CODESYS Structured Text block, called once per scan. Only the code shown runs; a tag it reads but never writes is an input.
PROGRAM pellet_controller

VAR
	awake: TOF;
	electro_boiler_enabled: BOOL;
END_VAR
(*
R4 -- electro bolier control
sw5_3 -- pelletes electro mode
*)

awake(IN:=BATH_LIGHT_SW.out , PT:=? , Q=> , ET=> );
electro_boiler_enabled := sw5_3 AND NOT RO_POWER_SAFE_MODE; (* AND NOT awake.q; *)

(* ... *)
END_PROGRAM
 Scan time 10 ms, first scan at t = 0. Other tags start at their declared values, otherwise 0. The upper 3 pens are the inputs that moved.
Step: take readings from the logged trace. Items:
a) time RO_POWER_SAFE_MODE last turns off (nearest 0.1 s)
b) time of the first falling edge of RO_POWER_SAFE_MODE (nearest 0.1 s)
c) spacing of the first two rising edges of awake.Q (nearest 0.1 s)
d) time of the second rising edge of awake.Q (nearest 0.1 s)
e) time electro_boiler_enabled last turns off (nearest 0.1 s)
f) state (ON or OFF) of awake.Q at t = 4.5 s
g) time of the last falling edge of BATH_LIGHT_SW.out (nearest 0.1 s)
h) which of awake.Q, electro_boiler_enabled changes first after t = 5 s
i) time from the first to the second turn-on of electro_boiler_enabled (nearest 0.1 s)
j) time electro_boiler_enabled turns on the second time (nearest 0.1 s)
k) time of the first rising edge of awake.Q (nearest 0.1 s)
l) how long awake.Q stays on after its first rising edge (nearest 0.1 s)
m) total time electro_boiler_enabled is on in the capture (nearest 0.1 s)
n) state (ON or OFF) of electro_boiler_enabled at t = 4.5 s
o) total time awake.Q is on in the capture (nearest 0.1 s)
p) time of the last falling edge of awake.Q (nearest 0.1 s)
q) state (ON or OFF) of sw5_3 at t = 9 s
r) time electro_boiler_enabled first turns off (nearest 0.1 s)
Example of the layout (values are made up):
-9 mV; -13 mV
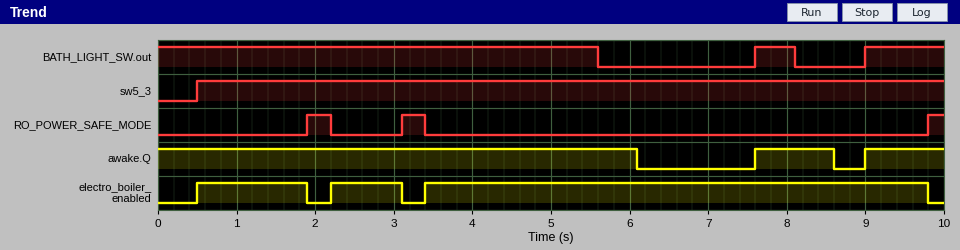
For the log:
3.4 s; 2.2 s; 1.4 s; 9.0 s; 9.8 s; ON; 8.1 s; awake.Q; 1.7 s; 2.2 s; 7.6 s; 1.0 s; 8.7 s; ON; 8.1 s; 8.6 s; ON; 1.9 s
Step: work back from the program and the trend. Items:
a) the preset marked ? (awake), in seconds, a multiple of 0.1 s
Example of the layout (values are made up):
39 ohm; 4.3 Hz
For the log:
0.5 s
